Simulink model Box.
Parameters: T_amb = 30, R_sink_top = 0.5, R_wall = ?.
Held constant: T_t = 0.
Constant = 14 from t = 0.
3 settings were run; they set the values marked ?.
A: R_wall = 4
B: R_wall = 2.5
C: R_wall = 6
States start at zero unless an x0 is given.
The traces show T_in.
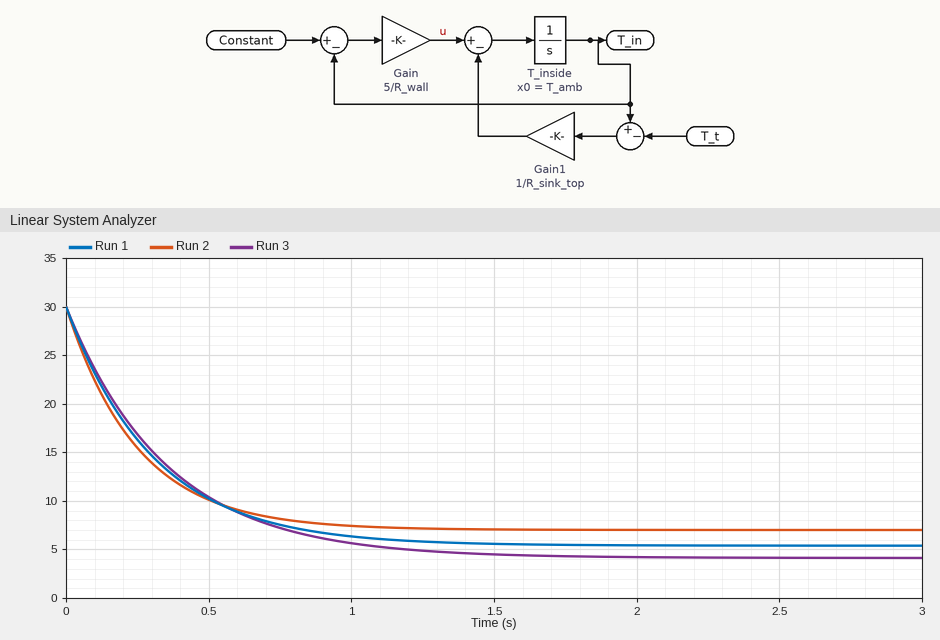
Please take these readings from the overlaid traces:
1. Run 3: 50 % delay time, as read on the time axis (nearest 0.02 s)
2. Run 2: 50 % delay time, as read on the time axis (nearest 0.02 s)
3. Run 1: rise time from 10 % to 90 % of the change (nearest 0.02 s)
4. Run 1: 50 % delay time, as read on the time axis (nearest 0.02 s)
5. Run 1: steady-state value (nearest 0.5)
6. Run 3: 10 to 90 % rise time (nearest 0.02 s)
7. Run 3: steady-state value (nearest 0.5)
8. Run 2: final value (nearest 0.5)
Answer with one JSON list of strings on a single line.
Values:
["0.24 s", "0.18 s", "0.68 s", "0.22 s", "5.5", "0.78 s", "4.0", "7.0"]
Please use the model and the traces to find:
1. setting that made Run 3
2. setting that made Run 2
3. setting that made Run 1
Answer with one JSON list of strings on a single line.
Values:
["C", "B", "A"]
